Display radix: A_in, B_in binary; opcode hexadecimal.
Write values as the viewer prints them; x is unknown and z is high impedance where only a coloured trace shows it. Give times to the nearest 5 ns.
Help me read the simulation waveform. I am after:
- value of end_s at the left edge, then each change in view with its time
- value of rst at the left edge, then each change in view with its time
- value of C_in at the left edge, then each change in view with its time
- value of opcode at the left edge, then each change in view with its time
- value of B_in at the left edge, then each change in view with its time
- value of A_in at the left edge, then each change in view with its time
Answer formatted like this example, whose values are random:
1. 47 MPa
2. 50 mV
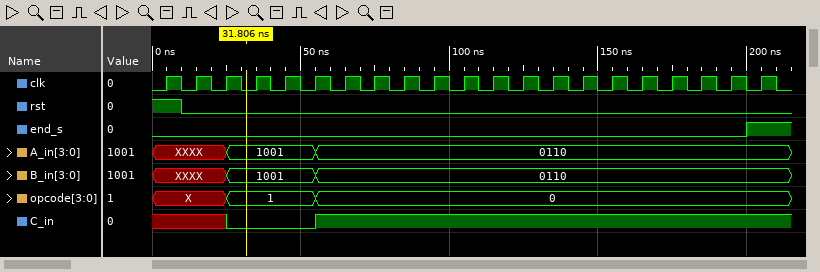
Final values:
1. 0, 1 at 200 ns
2. 1, 0 at 10 ns
3. x, 0 at 25 ns, 1 at 55 ns
4. X, 1 at 25 ns, 0 at 55 ns
5. XXXX, 1001 at 25 ns, 0110 at 55 ns
6. XXXX, 1001 at 25 ns, 0110 at 55 ns
